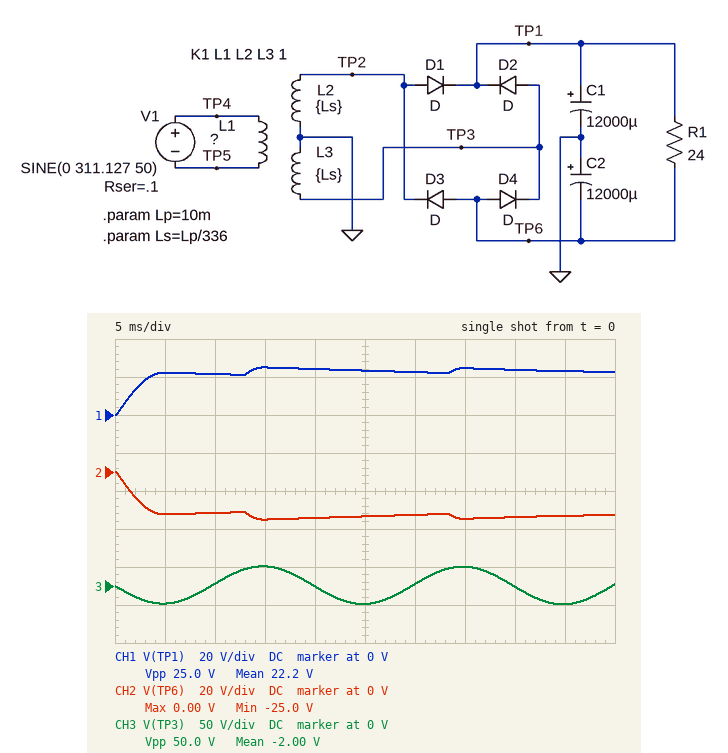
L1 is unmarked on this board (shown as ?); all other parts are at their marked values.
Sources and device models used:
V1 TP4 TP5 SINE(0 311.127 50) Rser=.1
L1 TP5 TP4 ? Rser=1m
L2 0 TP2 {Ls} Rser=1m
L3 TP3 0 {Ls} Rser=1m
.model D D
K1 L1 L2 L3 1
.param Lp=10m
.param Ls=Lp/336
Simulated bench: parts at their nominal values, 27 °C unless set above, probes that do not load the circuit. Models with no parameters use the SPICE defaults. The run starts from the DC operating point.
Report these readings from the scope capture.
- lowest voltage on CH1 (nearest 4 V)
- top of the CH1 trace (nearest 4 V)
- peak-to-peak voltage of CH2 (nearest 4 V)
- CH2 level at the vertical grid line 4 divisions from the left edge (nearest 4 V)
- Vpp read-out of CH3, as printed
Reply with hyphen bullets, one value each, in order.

- 0 V
- 24 V
- 24 V
- -24 V
- 50.0 V
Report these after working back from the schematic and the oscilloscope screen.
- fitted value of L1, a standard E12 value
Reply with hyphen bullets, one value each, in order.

- 4.7 mH
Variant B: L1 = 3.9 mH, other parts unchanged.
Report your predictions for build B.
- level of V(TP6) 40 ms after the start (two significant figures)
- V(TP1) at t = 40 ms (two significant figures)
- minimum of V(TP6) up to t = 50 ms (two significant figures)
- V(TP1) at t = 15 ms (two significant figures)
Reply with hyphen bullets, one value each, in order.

- -26 V
- 26 V
- -28 V
- 28 V
